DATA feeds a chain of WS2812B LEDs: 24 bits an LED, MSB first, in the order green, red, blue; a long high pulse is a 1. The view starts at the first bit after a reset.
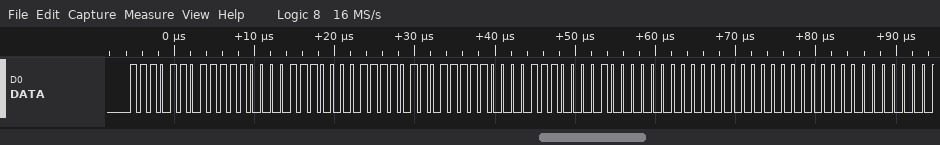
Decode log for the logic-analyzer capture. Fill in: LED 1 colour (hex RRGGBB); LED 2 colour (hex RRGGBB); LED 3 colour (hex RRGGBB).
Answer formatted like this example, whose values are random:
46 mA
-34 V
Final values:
#F0EDE1
#F0EDE1
#000000
